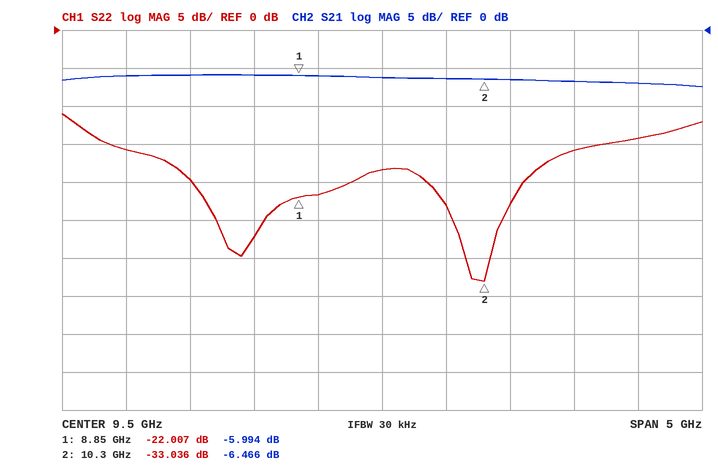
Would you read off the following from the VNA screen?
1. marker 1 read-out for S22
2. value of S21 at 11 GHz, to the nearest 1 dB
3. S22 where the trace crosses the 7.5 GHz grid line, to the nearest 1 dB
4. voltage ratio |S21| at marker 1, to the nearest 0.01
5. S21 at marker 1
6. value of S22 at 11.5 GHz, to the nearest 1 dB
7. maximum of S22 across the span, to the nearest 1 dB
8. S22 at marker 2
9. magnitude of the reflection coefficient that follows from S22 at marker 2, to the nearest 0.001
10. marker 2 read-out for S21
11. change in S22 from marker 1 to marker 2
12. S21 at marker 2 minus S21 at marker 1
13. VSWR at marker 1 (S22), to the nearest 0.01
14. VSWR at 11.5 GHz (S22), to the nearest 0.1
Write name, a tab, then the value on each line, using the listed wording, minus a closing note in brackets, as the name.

marker 1 read-out for S22	-22.007 dB
value of S21 at 11 GHz, to the nearest 1 dB	-7 dB
S22 where the trace crosses the 7.5 GHz grid line, to the nearest 1 dB	-16 dB
voltage ratio |S21| at marker 1, to the nearest 0.01	0.50
S21 at marker 1	-5.994 dB
value of S22 at 11.5 GHz, to the nearest 1 dB	-14 dB
maximum of S22 across the span, to the nearest 1 dB	-11 dB
S22 at marker 2	-33.036 dB
magnitude of the reflection coefficient that follows from S22 at marker 2, to the nearest 0.001	0.022
marker 2 read-out for S21	-6.466 dB
change in S22 from marker 1 to marker 2	-11.029 dB
S21 at marker 2 minus S21 at marker 1	-0.472 dB
VSWR at marker 1 (S22), to the nearest 0.01	1.17
VSWR at 11.5 GHz (S22), to the nearest 0.1	1.5
